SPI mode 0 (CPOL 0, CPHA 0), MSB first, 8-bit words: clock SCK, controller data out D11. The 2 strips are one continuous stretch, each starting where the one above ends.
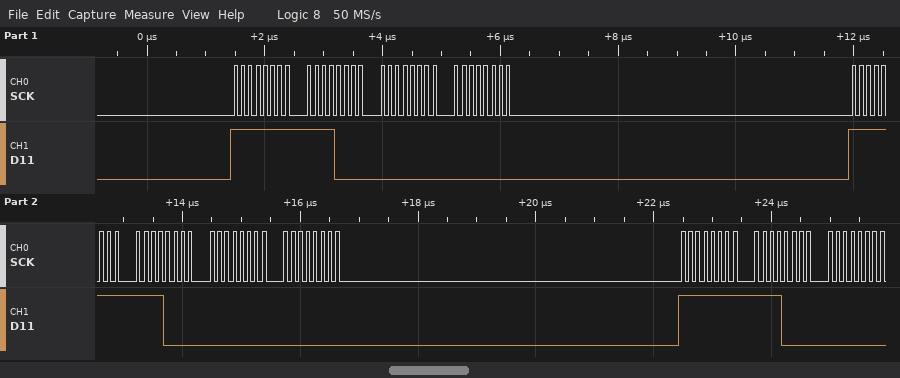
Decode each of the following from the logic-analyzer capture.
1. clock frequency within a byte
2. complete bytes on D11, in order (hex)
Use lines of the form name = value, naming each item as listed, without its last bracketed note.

clock frequency within a byte = 8 MHz
complete bytes on D11, in order = FF F0 00 00 FF F0 00 00 FF F0 00
